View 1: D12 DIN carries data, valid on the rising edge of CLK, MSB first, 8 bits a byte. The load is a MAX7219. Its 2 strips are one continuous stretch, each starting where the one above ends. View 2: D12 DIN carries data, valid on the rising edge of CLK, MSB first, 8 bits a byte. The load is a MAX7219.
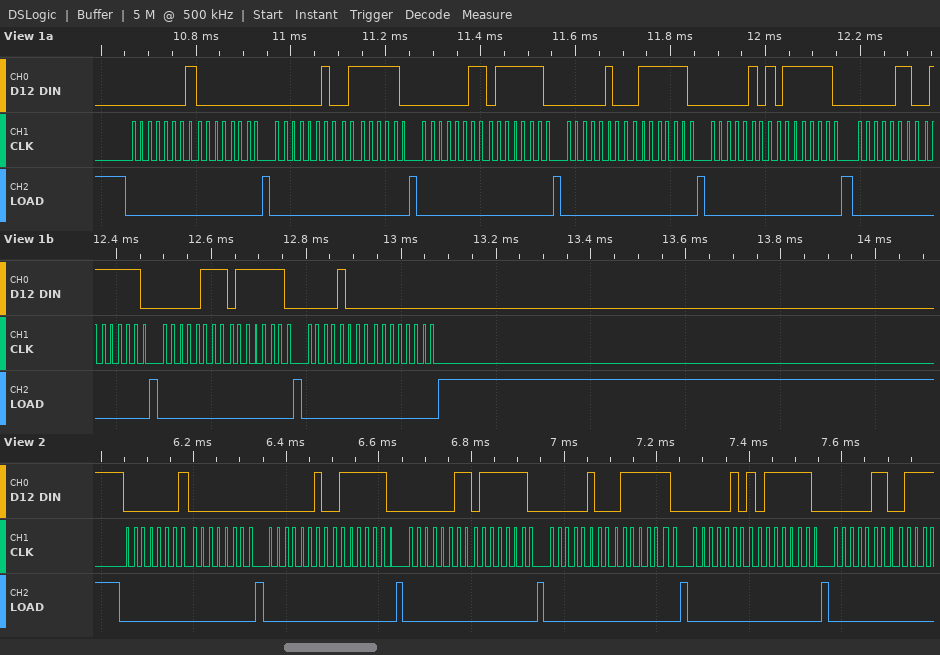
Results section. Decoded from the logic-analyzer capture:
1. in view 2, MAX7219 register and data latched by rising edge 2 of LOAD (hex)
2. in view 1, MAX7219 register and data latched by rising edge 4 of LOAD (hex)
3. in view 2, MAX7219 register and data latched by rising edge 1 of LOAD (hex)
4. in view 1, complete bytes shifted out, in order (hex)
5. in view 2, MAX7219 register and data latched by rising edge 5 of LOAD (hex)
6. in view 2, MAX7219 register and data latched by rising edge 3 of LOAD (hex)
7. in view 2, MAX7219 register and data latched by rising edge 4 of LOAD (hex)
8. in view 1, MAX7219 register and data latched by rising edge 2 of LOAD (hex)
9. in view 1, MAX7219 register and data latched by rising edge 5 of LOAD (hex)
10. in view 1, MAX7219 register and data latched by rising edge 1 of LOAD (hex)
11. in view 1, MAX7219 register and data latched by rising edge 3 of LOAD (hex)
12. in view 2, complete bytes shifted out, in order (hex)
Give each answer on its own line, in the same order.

register 0x2, data 0x7E
register 0x4, data 0x7E
register 0x1, data 0x00
01 00 02 7E 03 7E 04 7E 05 7E 06 7E 07 7E 08 00
register 0x5, data 0x7E
register 0x3, data 0x7E
register 0x4, data 0x7E
register 0x2, data 0x7E
register 0x5, data 0x7E
register 0x1, data 0x00
register 0x3, data 0x7E
01 00 02 7E 03 7E 04 7E 05 7E 06
